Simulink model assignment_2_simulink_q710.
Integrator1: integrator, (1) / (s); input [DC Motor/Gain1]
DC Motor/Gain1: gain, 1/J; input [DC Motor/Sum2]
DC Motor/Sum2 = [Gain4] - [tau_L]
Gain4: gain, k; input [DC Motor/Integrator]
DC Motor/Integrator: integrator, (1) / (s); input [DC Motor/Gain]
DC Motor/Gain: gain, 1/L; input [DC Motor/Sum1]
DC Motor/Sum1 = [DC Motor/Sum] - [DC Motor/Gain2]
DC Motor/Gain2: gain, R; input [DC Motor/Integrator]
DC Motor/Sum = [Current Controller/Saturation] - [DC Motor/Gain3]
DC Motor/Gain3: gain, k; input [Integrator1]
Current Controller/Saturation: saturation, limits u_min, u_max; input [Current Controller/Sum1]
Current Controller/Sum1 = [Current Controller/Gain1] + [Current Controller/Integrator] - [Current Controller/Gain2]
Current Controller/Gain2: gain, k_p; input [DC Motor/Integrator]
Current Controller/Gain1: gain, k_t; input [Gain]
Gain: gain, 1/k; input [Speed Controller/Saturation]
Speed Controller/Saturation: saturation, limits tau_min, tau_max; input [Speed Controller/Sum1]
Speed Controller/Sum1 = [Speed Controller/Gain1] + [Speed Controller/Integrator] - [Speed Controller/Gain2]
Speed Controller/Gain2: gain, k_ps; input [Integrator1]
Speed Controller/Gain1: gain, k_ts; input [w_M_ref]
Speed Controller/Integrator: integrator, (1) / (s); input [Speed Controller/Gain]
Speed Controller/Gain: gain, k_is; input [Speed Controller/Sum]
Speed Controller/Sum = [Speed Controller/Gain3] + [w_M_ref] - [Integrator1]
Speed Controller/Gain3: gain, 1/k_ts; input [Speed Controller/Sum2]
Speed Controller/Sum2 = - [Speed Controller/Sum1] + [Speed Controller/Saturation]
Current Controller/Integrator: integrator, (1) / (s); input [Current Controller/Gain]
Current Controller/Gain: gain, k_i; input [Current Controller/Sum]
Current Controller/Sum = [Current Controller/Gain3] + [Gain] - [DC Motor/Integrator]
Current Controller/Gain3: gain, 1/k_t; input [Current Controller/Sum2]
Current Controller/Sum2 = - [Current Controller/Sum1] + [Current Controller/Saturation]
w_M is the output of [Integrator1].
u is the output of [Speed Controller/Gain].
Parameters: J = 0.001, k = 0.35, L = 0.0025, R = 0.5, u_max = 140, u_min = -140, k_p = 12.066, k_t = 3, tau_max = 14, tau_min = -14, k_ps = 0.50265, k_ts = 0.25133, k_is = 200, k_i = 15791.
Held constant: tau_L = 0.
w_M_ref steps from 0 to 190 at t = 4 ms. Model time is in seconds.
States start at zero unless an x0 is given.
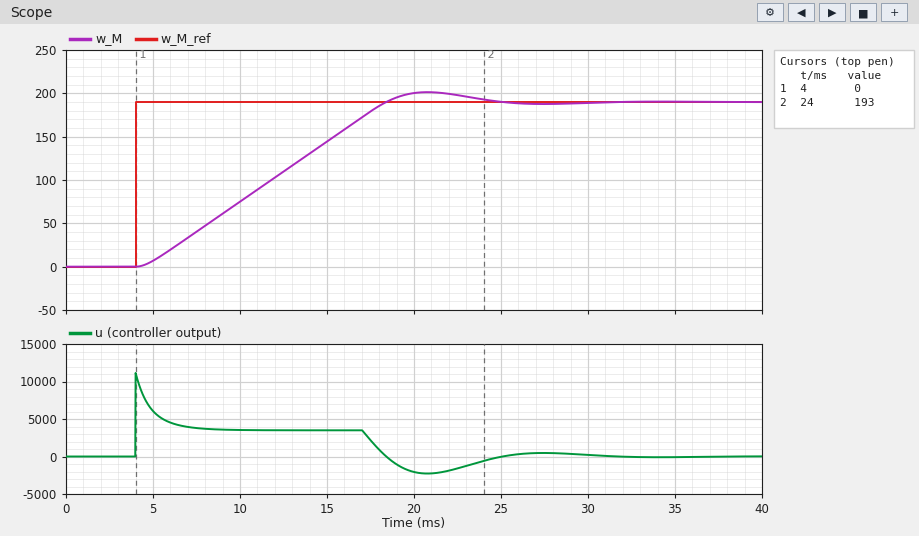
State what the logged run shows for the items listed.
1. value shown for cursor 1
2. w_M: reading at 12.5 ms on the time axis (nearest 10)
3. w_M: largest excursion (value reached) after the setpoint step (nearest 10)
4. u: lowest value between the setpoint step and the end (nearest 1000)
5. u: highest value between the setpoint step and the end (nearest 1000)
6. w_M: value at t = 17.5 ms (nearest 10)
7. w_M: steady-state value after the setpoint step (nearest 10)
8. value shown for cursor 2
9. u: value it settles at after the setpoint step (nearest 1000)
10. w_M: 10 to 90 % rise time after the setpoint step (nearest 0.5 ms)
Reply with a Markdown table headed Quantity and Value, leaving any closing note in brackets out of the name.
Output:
| Quantity | Value |
|---|---|
| value shown for cursor 1 | 0 |
| w_M: reading at 12.5 ms on the time axis | 110 |
| w_M: largest excursion (value reached) after the setpoint step | 200 |
| u: lowest value between the setpoint step and the end | -2000 |
| u: highest value between the setpoint step and the end | 11000 |
| w_M: value at t = 17.5 ms | 180 |
| w_M: steady-state value after the setpoint step | 190 |
| value shown for cursor 2 | 193 |
| u: value it settles at after the setpoint step | 0 |
| w_M: 10 to 90 % rise time after the setpoint step | 11.0 ms |
